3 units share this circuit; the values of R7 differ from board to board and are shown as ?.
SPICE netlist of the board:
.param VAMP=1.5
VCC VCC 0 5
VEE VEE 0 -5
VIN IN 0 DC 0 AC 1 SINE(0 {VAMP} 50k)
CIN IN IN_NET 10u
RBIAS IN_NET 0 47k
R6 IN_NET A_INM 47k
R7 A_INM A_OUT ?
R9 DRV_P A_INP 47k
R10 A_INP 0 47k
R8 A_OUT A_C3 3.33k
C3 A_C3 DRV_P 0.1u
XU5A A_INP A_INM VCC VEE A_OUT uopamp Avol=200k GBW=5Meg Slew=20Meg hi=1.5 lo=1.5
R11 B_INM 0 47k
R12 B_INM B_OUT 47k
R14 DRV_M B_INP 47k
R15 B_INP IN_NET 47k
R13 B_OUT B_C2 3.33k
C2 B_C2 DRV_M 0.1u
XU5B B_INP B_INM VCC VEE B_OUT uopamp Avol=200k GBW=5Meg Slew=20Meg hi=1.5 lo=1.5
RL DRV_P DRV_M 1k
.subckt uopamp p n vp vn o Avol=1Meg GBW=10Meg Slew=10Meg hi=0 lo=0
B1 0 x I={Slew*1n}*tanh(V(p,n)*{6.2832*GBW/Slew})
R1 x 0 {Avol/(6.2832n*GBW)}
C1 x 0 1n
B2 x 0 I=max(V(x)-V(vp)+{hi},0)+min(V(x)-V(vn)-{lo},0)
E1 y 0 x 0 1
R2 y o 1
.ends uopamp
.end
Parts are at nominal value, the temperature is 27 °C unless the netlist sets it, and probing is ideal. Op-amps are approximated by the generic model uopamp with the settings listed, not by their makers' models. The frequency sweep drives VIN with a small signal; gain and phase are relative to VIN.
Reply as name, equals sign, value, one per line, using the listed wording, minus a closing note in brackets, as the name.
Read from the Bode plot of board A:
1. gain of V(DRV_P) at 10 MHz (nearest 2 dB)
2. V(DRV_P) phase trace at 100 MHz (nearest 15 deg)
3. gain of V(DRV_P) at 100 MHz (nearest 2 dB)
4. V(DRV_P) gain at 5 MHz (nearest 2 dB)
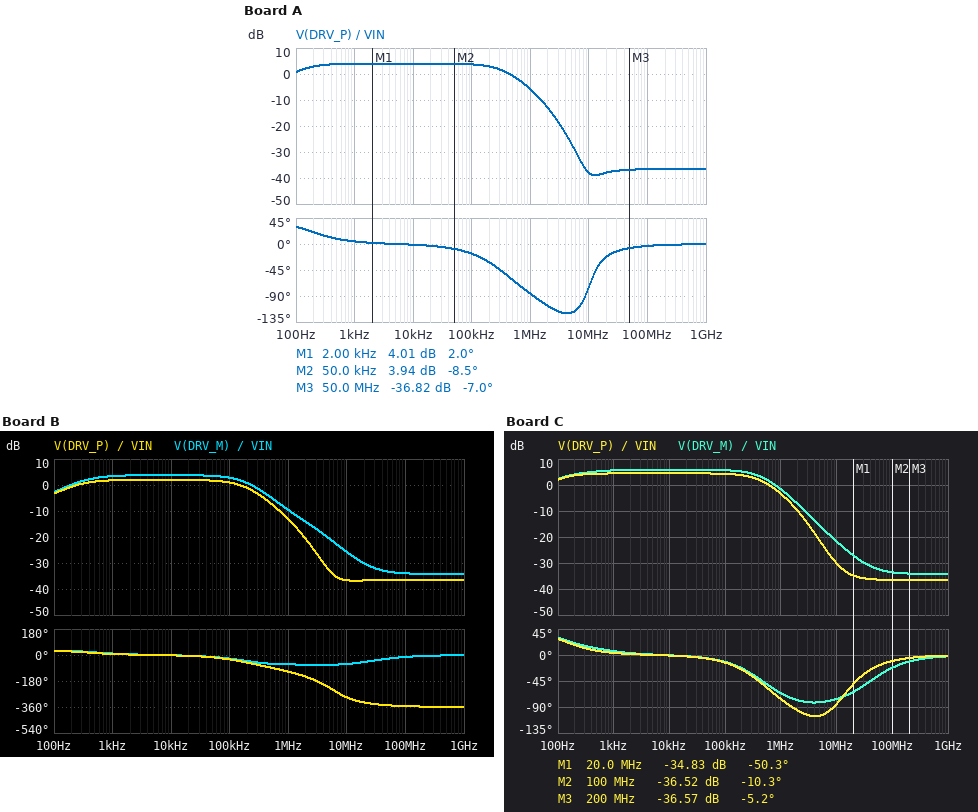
gain of V(DRV_P) at 10 MHz = -38 dB
V(DRV_P) phase trace at 100 MHz = 0 deg
gain of V(DRV_P) at 100 MHz = -36 dB
V(DRV_P) gain at 5 MHz = -26 dB
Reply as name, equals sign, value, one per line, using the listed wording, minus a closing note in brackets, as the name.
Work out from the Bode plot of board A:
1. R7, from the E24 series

R7, from the E24 series = 27 kΩ
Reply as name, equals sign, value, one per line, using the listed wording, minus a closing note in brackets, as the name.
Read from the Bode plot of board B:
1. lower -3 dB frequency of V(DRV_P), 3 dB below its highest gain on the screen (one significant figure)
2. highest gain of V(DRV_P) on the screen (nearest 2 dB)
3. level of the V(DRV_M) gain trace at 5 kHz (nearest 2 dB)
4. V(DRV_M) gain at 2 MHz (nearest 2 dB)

lower -3 dB frequency of V(DRV_P), 3 dB below its highest gain on the screen = 200 Hz
highest gain of V(DRV_P) on the screen = 2 dB
level of the V(DRV_M) gain trace at 5 kHz = 4 dB
V(DRV_M) gain at 2 MHz = -14 dB
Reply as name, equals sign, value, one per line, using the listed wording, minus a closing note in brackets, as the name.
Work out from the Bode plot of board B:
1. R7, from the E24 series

R7, from the E24 series = 39 kΩ
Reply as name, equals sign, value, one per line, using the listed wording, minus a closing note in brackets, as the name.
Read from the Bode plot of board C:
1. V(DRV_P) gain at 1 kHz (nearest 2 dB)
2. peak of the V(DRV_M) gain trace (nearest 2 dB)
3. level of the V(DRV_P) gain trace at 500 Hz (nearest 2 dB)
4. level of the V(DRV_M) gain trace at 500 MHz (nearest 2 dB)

V(DRV_P) gain at 1 kHz = 4 dB
peak of the V(DRV_M) gain trace = 6 dB
level of the V(DRV_P) gain trace at 500 Hz = 4 dB
level of the V(DRV_M) gain trace at 500 MHz = -34 dB
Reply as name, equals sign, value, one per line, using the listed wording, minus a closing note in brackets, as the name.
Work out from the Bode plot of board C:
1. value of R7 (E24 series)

value of R7 = 20 kΩ
